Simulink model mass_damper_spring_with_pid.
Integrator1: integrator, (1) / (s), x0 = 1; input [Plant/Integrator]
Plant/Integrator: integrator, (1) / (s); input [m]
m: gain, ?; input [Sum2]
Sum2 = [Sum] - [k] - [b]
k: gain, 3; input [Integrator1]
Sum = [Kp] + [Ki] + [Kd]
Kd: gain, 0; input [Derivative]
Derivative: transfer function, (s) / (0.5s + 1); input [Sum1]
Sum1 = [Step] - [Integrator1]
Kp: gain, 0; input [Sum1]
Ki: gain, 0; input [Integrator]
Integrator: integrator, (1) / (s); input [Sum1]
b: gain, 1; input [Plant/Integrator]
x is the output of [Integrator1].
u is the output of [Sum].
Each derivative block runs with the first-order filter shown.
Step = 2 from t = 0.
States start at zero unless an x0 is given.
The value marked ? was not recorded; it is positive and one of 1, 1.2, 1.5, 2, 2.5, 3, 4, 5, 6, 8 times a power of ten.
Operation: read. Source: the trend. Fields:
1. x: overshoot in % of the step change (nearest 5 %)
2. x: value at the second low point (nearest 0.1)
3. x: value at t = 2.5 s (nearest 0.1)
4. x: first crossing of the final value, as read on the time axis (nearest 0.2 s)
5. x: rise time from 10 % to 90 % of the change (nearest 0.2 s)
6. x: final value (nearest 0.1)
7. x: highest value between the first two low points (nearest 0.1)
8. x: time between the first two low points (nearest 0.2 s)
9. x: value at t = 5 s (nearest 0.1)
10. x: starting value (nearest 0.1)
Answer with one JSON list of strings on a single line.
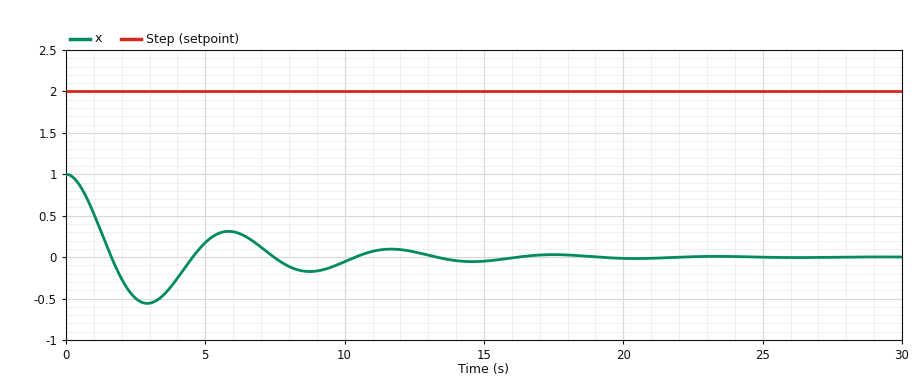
["55 %", "-0.2", "-0.5", "1.6 s", "1.0 s", "0.0", "0.3", "5.8 s", "0.2", "1.0"]
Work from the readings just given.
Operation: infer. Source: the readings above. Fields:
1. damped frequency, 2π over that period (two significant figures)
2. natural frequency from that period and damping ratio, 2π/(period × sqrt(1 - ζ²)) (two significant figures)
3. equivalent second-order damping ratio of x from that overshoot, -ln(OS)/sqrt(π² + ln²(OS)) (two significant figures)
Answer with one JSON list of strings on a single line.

["1.1 rad/s", "1.1 rad/s", "0.19"]
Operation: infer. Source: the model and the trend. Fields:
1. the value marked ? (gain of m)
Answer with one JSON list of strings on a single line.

["0.4"]
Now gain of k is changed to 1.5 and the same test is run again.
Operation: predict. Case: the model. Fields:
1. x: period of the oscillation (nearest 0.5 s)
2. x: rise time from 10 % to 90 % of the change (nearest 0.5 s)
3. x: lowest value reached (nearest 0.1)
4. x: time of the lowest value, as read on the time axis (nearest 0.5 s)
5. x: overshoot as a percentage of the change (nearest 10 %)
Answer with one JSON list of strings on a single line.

["8.5 s", "1.5 s", "-0.4", "4.0 s", "40 %"]
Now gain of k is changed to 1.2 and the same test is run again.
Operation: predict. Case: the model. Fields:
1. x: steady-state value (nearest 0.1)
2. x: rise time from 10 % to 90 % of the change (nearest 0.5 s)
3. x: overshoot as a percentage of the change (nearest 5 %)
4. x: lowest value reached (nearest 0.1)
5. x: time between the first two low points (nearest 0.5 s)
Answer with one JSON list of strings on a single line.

["0.0", "2.0 s", "40 %", "-0.4", "9.5 s"]
